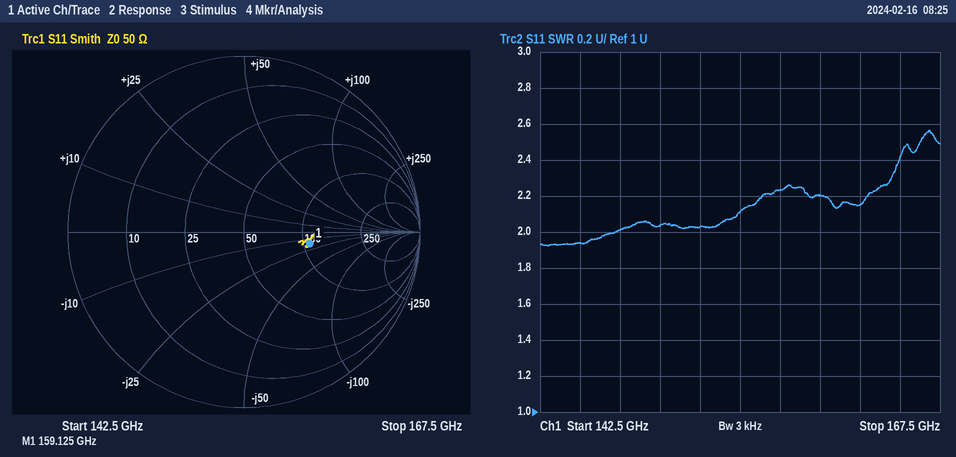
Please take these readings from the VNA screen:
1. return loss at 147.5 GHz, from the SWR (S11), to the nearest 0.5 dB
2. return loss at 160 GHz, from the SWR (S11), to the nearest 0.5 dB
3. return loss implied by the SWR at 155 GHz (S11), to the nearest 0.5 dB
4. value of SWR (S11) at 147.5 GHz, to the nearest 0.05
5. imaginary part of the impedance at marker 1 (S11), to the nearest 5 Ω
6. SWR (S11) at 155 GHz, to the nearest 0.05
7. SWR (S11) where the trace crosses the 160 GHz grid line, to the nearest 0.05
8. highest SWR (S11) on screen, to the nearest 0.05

9.5 dB
8.5 dB
9.0 dB
2.00
-15 Ω
2.10
2.20
2.55
